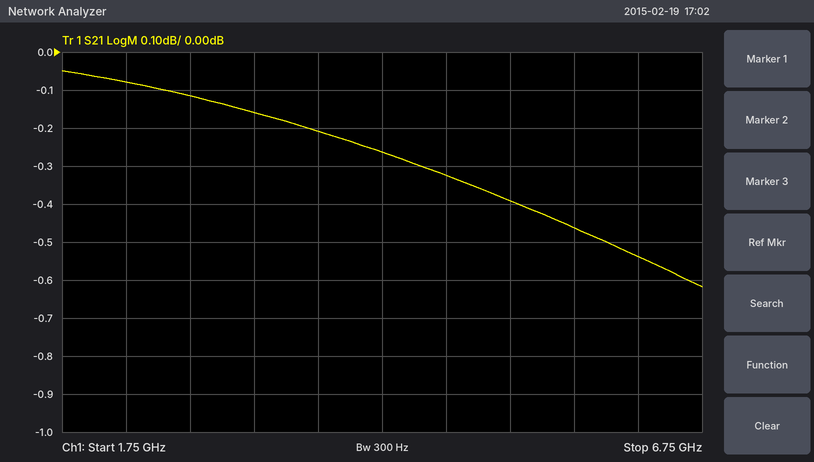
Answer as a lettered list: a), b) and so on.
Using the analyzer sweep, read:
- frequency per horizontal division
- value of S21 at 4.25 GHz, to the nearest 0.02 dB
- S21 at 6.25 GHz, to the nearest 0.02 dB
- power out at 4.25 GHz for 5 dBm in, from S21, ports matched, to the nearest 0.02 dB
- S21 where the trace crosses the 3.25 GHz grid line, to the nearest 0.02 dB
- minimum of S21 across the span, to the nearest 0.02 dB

a) 500 MHz
b) -0.26 dB
c) -0.54 dB
d) 4.74 dBm
e) -0.16 dB
f) -0.62 dB
